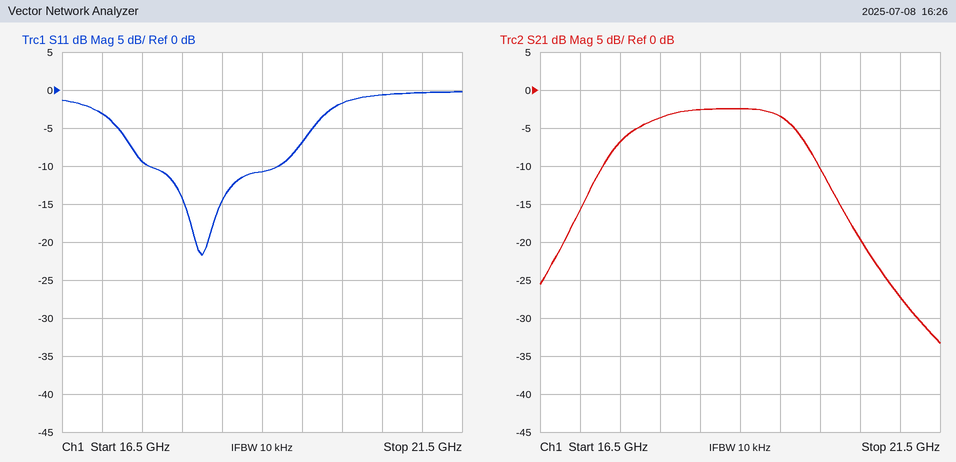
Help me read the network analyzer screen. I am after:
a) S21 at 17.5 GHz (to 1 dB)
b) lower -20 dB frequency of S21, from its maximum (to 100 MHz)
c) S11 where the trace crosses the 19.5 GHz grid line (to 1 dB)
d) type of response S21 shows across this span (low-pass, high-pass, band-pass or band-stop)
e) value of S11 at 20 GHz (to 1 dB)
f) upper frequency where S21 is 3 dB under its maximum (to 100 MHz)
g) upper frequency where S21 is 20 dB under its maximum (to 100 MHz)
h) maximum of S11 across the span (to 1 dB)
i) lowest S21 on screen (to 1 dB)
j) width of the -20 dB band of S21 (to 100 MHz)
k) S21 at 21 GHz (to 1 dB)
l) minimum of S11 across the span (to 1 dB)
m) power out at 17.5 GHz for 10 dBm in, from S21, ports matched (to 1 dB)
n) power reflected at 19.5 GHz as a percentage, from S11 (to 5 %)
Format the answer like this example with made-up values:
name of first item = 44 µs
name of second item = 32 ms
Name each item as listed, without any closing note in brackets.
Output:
S21 at 17.5 GHz = -7 dB
lower -20 dB frequency of S21, from its maximum = 16.7 GHz
S11 where the trace crosses the 19.5 GHz grid line = -7 dB
type of response S21 shows across this span = band-pass
value of S11 at 20 GHz = -2 dB
upper frequency where S21 is 3 dB under its maximum = 19.7 GHz
upper frequency where S21 is 20 dB under its maximum = 20.7 GHz
maximum of S11 across the span = 0 dB
lowest S21 on screen = -33 dB
width of the -20 dB band of S21 = 4.0 GHz
S21 at 21 GHz = -27 dB
minimum of S11 across the span = -22 dB
power out at 17.5 GHz for 10 dBm in, from S21, ports matched = 3 dBm
power reflected at 19.5 GHz as a percentage, from S11 = 20 %
